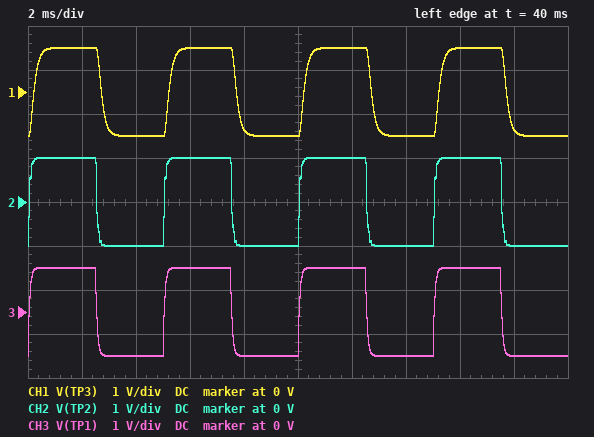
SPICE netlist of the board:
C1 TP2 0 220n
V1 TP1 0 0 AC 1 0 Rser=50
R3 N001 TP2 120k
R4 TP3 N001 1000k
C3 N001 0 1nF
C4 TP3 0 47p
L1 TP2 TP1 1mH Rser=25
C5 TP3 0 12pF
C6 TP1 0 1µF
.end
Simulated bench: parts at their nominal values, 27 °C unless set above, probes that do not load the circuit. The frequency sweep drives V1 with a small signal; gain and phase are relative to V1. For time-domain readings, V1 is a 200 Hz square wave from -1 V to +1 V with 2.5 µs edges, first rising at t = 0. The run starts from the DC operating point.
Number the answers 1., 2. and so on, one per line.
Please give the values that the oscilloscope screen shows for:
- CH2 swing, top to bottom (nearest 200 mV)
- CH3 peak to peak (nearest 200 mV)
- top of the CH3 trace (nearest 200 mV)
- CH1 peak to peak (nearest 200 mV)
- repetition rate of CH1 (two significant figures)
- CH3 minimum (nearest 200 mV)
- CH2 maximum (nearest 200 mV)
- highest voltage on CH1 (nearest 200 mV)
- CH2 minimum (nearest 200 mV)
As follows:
1. 2.0 V
2. 2.0 V
3. 1.0 V
4. 2.0 V
5. 200 Hz
6. -1.0 V
7. 1.0 V
8. 1.0 V
9. -1.0 V
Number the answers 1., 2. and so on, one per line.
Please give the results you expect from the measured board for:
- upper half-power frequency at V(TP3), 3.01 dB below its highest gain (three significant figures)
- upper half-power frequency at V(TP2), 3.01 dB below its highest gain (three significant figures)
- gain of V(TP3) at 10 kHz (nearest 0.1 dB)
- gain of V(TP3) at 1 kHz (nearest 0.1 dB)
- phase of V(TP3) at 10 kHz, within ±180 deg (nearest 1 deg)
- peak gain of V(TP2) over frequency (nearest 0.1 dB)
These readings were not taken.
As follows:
1. 946 Hz
2. 2.88 kHz
3. -34.2 dB
4. -3.3 dB
5. 80 deg
6. 0 dB
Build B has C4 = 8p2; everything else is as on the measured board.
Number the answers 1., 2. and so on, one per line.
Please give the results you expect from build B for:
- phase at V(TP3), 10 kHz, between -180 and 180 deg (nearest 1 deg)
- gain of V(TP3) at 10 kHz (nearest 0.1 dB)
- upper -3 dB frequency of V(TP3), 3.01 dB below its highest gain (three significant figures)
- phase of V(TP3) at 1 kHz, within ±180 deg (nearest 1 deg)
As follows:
1. 103 deg
2. -26.7 dB
3. 1.08 kHz
4. -68 deg
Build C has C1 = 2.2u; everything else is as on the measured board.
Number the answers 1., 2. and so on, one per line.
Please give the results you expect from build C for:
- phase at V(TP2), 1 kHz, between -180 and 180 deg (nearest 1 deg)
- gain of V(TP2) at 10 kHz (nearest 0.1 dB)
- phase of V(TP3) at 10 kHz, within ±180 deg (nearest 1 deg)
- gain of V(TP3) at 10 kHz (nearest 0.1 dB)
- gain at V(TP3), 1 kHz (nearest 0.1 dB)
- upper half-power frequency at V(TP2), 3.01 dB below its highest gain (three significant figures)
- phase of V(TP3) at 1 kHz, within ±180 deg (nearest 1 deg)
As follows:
1. -59 deg
2. -27.3 dB
3. -13 deg
4. -56.6 dB
5. -6.6 dB
6. 842 Hz
7. -117 deg
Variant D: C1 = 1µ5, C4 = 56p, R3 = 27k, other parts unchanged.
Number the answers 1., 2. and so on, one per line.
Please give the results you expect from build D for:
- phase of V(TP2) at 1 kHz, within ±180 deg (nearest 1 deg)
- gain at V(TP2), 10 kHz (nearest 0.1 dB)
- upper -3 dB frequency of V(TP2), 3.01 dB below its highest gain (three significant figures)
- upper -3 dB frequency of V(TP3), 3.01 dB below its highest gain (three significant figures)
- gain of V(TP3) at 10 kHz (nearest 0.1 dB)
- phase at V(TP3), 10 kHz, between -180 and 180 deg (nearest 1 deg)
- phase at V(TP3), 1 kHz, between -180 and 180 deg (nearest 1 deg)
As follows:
1. -49 deg
2. -23.5 dB
3. 1.15 kHz
4. 936 Hz
5. -42.3 dB
6. 10 deg
7. -82 deg
